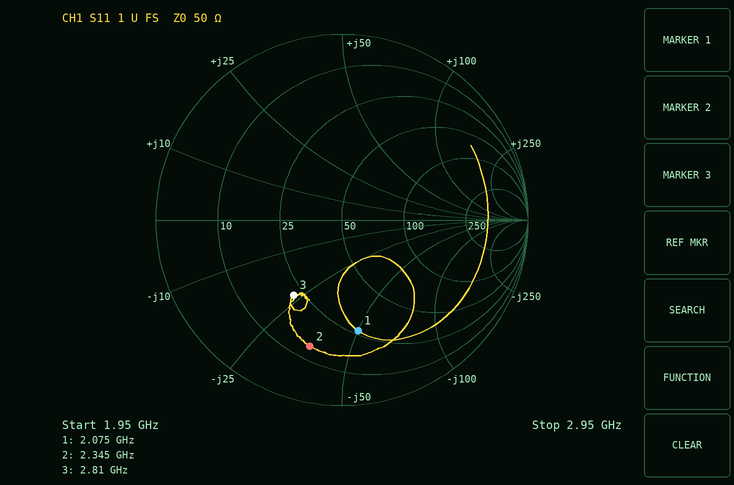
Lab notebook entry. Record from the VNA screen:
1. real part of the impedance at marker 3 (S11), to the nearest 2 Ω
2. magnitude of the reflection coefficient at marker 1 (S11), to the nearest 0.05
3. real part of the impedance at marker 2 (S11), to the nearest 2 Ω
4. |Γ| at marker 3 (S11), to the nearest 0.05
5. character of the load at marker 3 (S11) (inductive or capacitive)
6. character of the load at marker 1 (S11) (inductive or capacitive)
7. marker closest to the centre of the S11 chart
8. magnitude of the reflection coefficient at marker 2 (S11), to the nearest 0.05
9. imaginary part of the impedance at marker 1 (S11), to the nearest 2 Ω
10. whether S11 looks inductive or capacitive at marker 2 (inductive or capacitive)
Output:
22 Ω
0.60
14 Ω
0.50
capacitive
capacitive
marker 3
0.70
-50 Ω
capacitive
